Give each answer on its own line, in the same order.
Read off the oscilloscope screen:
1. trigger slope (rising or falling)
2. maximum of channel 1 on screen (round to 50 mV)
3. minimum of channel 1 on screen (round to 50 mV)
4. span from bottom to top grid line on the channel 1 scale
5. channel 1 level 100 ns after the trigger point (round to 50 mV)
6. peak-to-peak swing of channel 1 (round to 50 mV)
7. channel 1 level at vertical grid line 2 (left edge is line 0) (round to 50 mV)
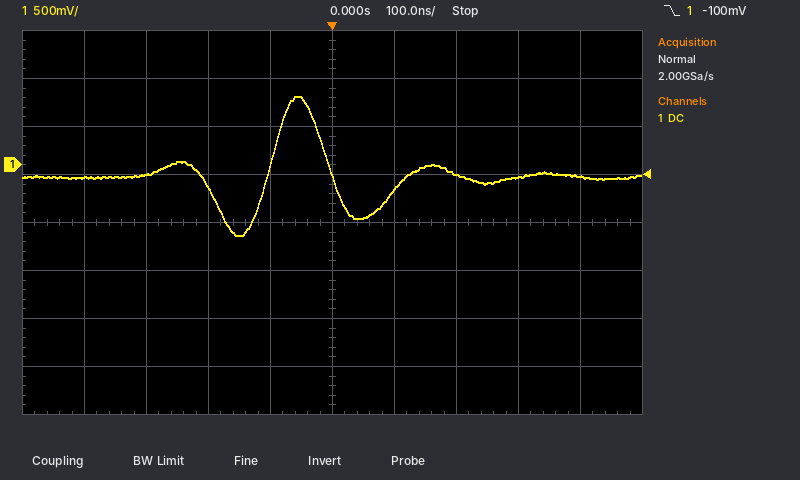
falling
700 mV
-750 mV
4 V
-250 mV
1.45 V
-100 mV
